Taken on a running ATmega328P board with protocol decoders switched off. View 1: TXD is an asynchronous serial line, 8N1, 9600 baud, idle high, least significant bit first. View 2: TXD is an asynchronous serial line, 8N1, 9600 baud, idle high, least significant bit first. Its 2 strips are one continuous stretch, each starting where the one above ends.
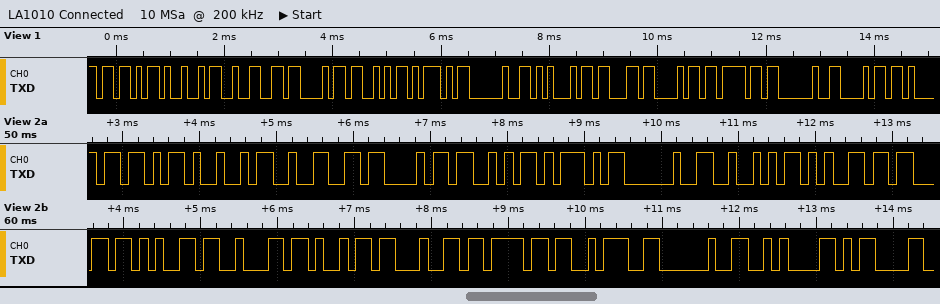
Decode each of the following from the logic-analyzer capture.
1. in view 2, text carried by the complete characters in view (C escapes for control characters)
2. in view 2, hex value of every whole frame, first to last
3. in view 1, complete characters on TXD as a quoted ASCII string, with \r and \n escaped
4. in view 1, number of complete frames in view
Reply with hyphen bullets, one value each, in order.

- "[I2CS] Recebido: \n\r"
- 5B 49 32 43 53 5D 20 52 65 63 65 62 69 64 6F 3A 20 0A 0D
- "[I2CS] Echo h"
- 13
